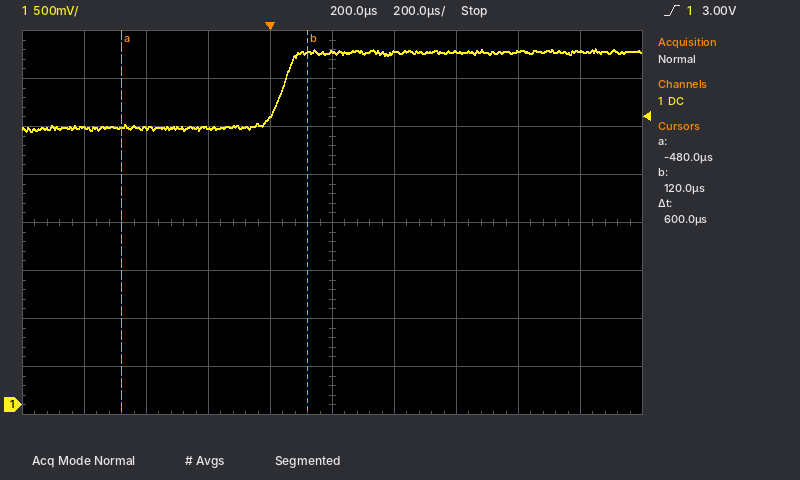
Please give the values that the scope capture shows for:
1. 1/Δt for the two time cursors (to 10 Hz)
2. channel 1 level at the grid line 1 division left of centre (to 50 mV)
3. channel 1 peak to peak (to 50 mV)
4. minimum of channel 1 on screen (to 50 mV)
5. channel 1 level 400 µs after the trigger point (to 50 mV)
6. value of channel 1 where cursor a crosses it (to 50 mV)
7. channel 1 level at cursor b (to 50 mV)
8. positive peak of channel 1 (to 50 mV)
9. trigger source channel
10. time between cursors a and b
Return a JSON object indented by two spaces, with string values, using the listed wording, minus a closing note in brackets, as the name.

{
  "1/Δt for the two time cursors": "1.67 kHz",
  "channel 1 level at the grid line 1 division left of centre": "3.00 V",
  "channel 1 peak to peak": "850 mV",
  "minimum of channel 1 on screen": "2.85 V",
  "channel 1 level 400 µs after the trigger point": "3.65 V",
  "value of channel 1 where cursor a crosses it": "2.90 V",
  "channel 1 level at cursor b": "3.65 V",
  "positive peak of channel 1": "3.70 V",
  "trigger source channel": "channel 1",
  "time between cursors a and b": "600 µs"
}
